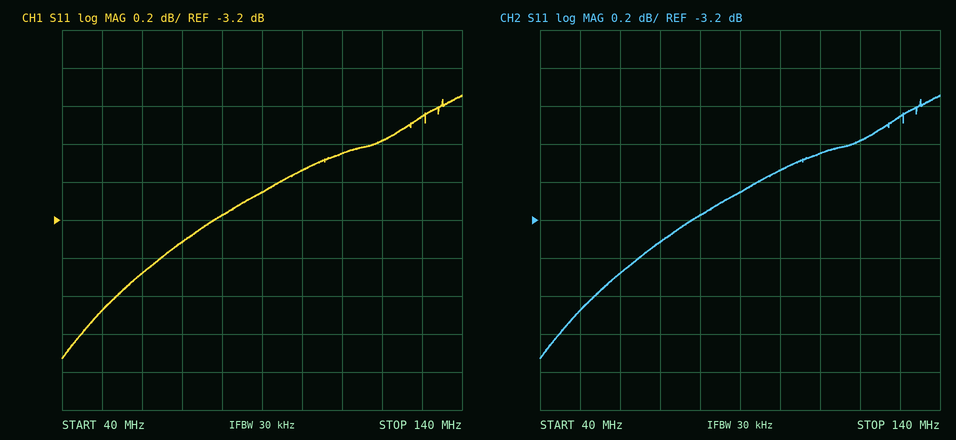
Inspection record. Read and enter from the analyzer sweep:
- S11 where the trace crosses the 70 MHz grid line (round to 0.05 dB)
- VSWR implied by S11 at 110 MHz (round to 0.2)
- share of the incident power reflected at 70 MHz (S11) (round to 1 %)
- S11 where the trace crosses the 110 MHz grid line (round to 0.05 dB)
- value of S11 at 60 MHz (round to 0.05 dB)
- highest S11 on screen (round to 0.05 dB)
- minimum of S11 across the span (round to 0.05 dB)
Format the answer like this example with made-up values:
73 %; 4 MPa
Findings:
-3.30 dB; 6.2; 47 %; -2.85 dB; -3.50 dB; -2.55 dB; -3.95 dB
